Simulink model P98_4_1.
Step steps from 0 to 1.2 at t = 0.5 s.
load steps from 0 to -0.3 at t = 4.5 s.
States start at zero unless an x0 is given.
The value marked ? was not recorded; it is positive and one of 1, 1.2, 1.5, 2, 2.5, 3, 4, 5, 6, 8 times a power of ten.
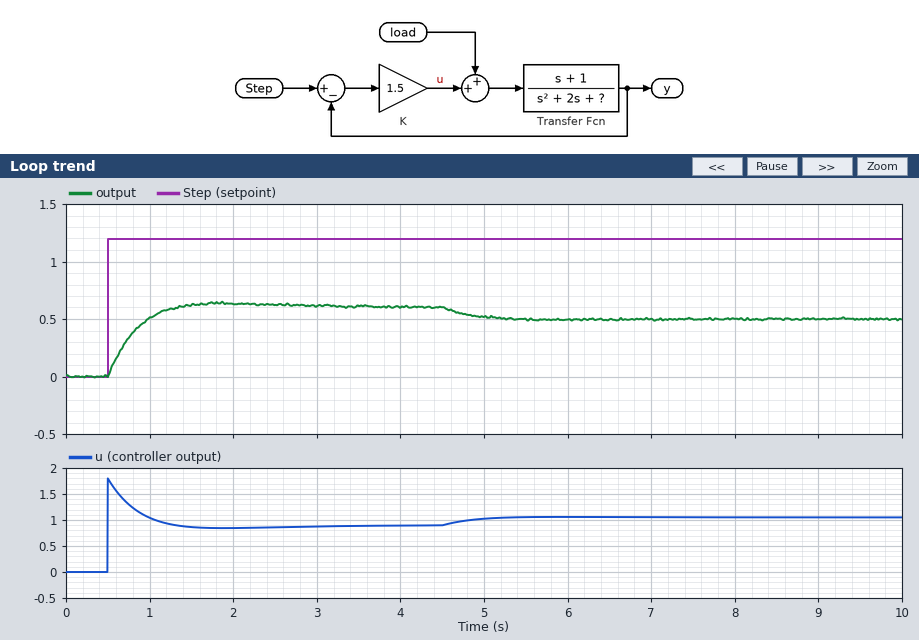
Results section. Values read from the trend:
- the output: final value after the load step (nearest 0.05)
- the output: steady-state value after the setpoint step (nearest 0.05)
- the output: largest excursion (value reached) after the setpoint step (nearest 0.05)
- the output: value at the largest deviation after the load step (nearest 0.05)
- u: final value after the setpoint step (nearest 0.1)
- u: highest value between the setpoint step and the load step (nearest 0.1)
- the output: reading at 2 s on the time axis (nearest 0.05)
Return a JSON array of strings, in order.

["0.50", "0.60", "0.65", "0.50", "0.9", "1.8", "0.65"]
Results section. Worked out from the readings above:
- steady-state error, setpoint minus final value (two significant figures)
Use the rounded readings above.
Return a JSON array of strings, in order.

["0.60"]
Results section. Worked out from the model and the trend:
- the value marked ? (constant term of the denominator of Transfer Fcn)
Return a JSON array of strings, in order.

["1.5"]
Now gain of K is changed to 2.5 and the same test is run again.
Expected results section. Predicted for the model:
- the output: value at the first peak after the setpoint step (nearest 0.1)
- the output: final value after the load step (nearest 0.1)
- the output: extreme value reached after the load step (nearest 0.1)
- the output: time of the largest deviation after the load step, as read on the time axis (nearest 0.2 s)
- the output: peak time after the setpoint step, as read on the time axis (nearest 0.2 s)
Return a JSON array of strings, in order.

["0.8", "0.7", "0.7", "5.6 s", "1.6 s"]
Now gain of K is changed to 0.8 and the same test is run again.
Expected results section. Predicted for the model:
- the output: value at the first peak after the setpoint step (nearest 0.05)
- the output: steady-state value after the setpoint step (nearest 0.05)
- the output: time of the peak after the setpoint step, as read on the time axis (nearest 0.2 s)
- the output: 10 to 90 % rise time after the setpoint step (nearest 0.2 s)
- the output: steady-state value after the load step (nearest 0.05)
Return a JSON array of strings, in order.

["0.45", "0.40", "2.2 s", "0.6 s", "0.30"]
